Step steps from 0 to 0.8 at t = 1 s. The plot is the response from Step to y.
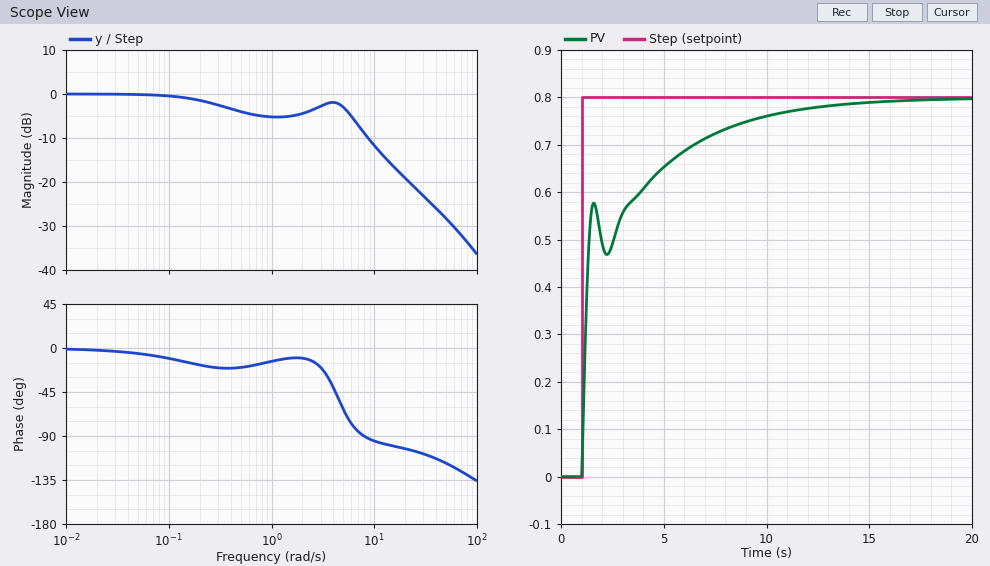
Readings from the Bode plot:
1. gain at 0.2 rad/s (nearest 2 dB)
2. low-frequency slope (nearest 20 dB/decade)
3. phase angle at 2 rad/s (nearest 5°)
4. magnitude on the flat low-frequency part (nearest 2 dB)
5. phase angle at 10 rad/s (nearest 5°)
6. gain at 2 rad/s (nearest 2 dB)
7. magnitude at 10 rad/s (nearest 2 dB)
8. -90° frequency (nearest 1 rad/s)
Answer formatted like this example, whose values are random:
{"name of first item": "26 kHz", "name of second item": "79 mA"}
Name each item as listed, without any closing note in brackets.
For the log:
{"gain at 0.2 rad/s": "-2 dB", "low-frequency slope": "0 dB/decade", "phase angle at 2 rad/s": "-10°", "magnitude on the flat low-frequency part": "0 dB", "phase angle at 10 rad/s": "-95°", "gain at 2 rad/s": "-4 dB", "magnitude at 10 rad/s": "-12 dB", "-90° frequency": "8 rad/s"}
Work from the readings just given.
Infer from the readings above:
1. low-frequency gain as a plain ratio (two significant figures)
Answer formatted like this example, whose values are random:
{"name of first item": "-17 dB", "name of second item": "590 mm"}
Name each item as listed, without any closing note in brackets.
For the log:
{"low-frequency gain as a plain ratio": "1.0"}
